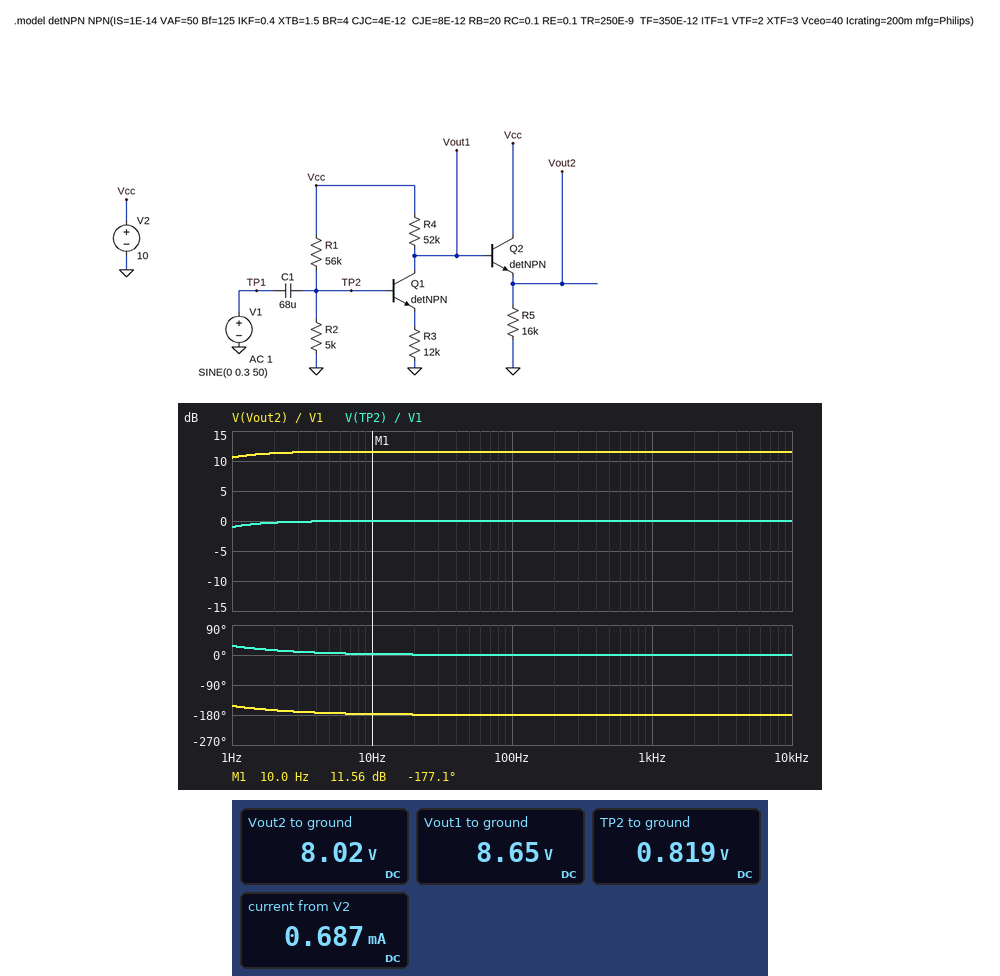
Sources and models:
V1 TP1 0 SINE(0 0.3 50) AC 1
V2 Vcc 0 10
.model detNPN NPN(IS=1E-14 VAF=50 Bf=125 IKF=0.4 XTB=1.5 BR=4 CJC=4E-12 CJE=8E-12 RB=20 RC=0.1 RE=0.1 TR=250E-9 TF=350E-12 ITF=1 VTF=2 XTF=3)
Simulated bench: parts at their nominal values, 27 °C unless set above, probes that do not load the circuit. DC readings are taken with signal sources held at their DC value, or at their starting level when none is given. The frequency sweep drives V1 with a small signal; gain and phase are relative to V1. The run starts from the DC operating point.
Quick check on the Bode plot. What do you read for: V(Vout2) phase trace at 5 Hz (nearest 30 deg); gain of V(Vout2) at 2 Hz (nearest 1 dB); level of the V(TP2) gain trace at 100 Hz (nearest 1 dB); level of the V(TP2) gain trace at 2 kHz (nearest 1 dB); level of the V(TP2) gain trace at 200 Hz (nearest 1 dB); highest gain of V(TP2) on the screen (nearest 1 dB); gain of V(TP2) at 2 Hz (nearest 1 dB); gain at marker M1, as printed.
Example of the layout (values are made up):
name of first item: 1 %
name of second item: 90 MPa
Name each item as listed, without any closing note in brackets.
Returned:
V(Vout2) phase trace at 5 Hz: -180 deg
gain of V(Vout2) at 2 Hz: 11 dB
level of the V(TP2) gain trace at 100 Hz: 0 dB
level of the V(TP2) gain trace at 2 kHz: 0 dB
level of the V(TP2) gain trace at 200 Hz: 0 dB
highest gain of V(TP2) on the screen: 0 dB
gain of V(TP2) at 2 Hz: 0 dB
gain at marker M1, as printed: 11.56 dB
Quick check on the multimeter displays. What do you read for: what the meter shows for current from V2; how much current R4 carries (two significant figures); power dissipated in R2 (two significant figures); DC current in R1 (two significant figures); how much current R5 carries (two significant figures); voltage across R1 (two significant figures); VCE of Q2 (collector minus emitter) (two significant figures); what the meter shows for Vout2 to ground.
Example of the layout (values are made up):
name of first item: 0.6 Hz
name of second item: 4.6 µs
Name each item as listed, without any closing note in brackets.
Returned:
what the meter shows for current from V2: 0.687 mA
how much current R4 carries: 26 µA
power dissipated in R2: 130 µW
DC current in R1: 160 µA
how much current R5 carries: 500 µA
voltage across R1: 9.2 V
VCE of Q2 (collector minus emitter): 2.0 V
what the meter shows for Vout2 to ground: 8.02 V
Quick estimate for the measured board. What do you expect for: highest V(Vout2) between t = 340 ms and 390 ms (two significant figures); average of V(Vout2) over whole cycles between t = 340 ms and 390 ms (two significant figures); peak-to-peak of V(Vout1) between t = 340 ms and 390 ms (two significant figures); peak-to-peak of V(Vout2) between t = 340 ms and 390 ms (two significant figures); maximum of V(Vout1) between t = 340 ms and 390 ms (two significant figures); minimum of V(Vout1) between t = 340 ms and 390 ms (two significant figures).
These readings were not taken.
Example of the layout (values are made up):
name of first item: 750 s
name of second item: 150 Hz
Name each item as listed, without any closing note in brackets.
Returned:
highest V(Vout2) between t = 340 ms and 390 ms: 9.0 V
average of V(Vout2) over whole cycles between t = 340 ms and 390 ms: 8.0 V
peak-to-peak of V(Vout1) between t = 340 ms and 390 ms: 2.2 V
peak-to-peak of V(Vout2) between t = 340 ms and 390 ms: 2.2 V
maximum of V(Vout1) between t = 340 ms and 390 ms: 9.7 V
minimum of V(Vout1) between t = 340 ms and 390 ms: 7.5 V
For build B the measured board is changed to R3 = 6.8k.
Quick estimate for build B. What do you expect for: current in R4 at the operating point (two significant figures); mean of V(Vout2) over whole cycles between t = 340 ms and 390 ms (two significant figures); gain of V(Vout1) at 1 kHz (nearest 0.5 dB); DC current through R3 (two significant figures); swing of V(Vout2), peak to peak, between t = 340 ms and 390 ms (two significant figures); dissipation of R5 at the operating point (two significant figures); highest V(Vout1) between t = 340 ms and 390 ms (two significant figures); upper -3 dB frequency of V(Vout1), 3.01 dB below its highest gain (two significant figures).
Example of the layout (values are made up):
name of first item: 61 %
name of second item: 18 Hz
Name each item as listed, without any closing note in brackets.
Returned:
current in R4 at the operating point: 40 µA
mean of V(Vout2) over whole cycles between t = 340 ms and 390 ms: 7.2 V
gain of V(Vout1) at 1 kHz: 16.5 dB
DC current through R3: 37 µA
swing of V(Vout2), peak to peak, between t = 340 ms and 390 ms: 3.8 V
dissipation of R5 at the operating point: 3.3 mW
highest V(Vout1) between t = 340 ms and 390 ms: 9.6 V
upper -3 dB frequency of V(Vout1), 3.01 dB below its highest gain: 710 kHz
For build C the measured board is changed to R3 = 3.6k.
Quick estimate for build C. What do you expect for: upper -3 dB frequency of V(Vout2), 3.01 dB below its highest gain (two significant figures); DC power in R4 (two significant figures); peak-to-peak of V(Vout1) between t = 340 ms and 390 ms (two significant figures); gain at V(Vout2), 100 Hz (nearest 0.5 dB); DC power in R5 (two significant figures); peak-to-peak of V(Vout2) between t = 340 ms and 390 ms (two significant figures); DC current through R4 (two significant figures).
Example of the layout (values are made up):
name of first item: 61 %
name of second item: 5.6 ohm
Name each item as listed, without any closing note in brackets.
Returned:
upper -3 dB frequency of V(Vout2), 3.01 dB below its highest gain: 730 kHz
DC power in R4: 240 µW
peak-to-peak of V(Vout1) between t = 340 ms and 390 ms: 7.0 V
gain at V(Vout2), 100 Hz: 22.0 dB
DC power in R5: 2.1 mW
peak-to-peak of V(Vout2) between t = 340 ms and 390 ms: 6.9 V
DC current through R4: 68 µA
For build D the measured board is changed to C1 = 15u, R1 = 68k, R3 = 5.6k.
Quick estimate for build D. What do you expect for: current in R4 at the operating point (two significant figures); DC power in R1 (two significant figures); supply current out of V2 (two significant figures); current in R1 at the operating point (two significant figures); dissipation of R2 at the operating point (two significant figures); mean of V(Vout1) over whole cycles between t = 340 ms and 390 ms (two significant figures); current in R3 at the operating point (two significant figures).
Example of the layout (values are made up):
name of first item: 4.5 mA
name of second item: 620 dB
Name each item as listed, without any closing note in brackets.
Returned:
current in R4 at the operating point: 27 µA
DC power in R1: 1.3 mW
supply current out of V2: 660 µA
current in R1 at the operating point: 140 µA
dissipation of R2 at the operating point: 94 µW
mean of V(Vout1) over whole cycles between t = 340 ms and 390 ms: 8.3 V
current in R3 at the operating point: 23 µA
